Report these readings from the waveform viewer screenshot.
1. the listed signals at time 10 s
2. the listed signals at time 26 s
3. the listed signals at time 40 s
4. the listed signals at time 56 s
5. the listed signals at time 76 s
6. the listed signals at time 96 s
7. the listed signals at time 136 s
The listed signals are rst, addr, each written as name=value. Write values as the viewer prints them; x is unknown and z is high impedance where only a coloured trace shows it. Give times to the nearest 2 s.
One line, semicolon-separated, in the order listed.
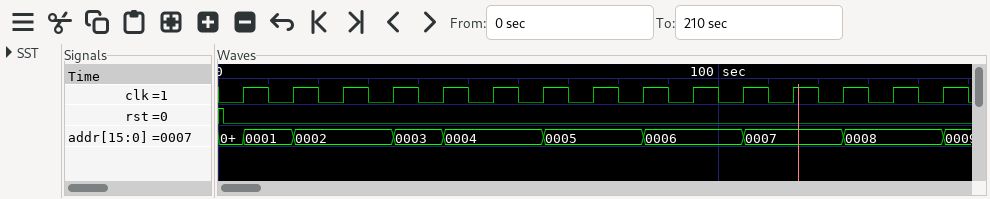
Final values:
rst=0, addr=0001; rst=0, addr=0002; rst=0, addr=0003; rst=0, addr=0004; rst=0, addr=0005; rst=0, addr=0006; rst=0, addr=0008
